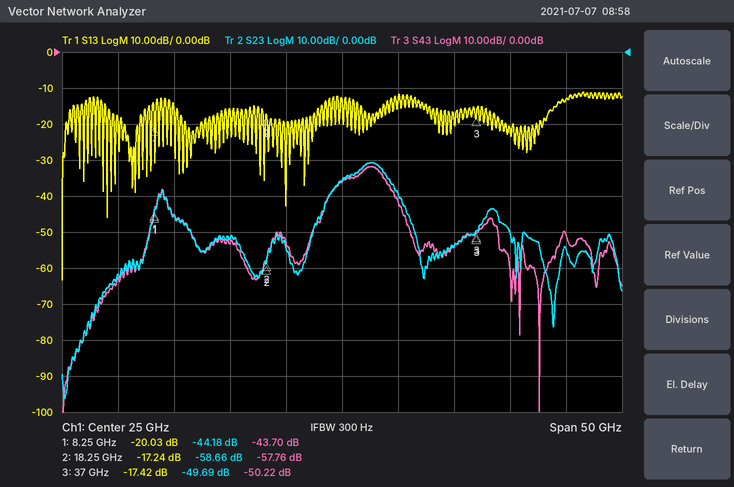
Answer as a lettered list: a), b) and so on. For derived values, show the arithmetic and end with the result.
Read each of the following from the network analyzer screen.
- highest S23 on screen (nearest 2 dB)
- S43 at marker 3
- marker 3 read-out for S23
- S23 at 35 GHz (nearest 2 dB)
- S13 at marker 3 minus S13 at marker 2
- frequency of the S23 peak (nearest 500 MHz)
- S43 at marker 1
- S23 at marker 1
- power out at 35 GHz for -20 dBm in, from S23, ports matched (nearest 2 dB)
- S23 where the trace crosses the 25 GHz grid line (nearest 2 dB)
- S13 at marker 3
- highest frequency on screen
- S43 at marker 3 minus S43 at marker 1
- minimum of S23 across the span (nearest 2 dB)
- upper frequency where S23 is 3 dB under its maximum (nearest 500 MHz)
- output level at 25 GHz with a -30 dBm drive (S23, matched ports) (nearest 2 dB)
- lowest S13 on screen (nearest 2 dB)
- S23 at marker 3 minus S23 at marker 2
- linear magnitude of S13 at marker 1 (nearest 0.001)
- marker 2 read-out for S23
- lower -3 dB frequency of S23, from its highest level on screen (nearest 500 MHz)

a) -30 dB
b) -50.22 dB
c) -49.69 dB
d) -54 dB
e) -17.42 − (-17.24) = -0.18 dB
f) 27.5 GHz
g) -43.70 dB
h) -44.18 dB
i) -20 dBm + (-54 dB) = -74 dBm
j) -36 dB
k) -17.42 dB
l) 50 GHz
m) -50.22 − (-43.7) = -6.52 dB
n) -96 dB
o) 29.0 GHz
p) -30 dBm + (-36 dB) = -66 dBm
q) -64 dB
r) -49.69 − (-58.66) = 8.97 dB
s) 10^(-20.03/20) ≈ 0.100
t) -58.66 dB
u) 26.0 GHz
